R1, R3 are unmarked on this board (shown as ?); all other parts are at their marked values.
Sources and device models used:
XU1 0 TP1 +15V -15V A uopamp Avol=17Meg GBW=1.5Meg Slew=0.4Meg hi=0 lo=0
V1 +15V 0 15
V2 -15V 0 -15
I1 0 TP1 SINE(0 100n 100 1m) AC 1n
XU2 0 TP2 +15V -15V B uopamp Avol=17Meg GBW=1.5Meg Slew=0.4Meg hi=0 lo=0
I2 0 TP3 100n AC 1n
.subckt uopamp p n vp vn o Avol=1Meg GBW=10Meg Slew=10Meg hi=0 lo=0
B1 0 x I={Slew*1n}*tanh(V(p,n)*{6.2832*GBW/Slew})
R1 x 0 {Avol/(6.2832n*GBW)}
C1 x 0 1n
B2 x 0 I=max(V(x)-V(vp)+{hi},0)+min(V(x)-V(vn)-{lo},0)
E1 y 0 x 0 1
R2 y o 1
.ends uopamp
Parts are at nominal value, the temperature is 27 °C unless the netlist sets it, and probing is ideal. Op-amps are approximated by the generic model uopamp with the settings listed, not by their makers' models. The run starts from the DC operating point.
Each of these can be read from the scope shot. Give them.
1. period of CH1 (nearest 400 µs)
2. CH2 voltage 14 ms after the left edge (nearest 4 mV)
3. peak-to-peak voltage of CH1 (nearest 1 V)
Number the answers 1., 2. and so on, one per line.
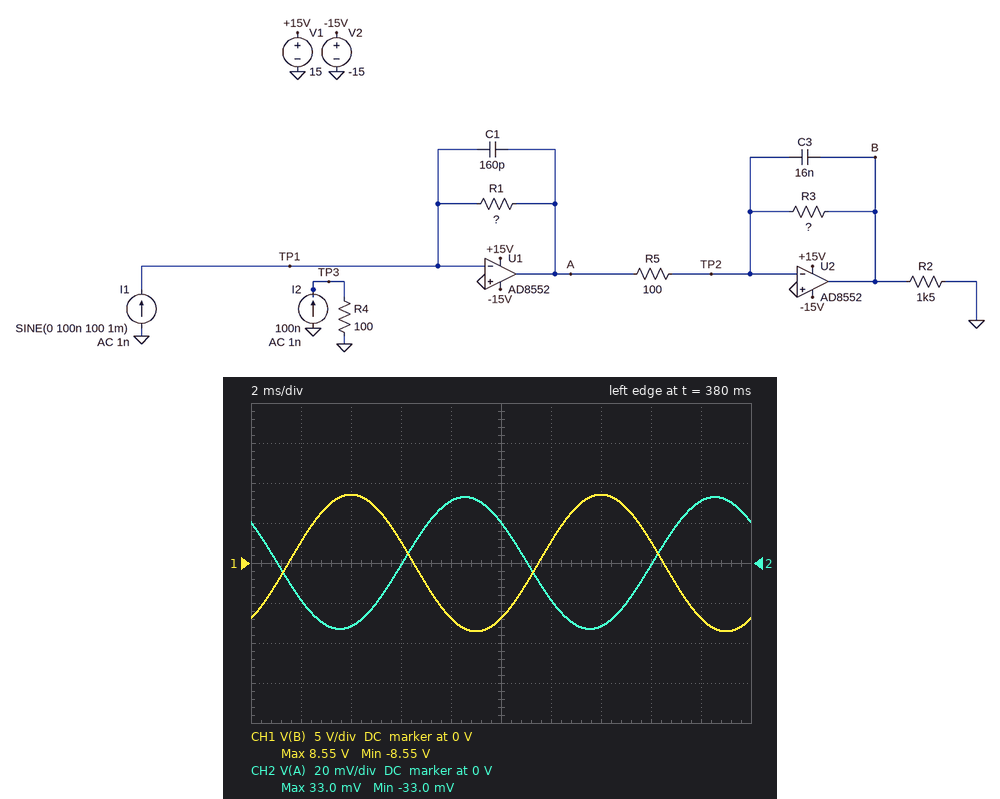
1. 10.0 ms
2. -32 mV
3. 17 V
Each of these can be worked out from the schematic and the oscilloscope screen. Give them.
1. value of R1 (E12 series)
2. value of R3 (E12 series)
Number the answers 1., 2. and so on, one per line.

1. 330 kΩ
2. 27 kΩ
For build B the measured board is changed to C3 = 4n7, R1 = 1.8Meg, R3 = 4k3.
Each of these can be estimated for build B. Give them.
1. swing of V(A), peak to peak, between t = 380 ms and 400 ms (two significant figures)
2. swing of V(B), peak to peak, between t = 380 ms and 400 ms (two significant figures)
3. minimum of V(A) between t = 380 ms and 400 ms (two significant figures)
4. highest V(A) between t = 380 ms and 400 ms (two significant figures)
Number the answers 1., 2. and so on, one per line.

1. 350 mV
2. 15 V
3. -180 mV
4. 180 mV
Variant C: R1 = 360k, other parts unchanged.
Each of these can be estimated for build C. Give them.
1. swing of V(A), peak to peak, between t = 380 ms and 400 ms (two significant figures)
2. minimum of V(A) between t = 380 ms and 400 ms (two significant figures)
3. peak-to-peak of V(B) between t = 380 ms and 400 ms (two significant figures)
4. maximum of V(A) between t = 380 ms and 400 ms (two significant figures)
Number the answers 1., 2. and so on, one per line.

1. 72 mV
2. -36 mV
3. 19 V
4. 36 mV
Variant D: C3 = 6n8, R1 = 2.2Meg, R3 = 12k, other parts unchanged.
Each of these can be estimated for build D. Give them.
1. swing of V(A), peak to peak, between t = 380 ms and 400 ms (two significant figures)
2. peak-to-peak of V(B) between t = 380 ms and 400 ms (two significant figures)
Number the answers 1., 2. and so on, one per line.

1. 430 mV
2. 30 V
